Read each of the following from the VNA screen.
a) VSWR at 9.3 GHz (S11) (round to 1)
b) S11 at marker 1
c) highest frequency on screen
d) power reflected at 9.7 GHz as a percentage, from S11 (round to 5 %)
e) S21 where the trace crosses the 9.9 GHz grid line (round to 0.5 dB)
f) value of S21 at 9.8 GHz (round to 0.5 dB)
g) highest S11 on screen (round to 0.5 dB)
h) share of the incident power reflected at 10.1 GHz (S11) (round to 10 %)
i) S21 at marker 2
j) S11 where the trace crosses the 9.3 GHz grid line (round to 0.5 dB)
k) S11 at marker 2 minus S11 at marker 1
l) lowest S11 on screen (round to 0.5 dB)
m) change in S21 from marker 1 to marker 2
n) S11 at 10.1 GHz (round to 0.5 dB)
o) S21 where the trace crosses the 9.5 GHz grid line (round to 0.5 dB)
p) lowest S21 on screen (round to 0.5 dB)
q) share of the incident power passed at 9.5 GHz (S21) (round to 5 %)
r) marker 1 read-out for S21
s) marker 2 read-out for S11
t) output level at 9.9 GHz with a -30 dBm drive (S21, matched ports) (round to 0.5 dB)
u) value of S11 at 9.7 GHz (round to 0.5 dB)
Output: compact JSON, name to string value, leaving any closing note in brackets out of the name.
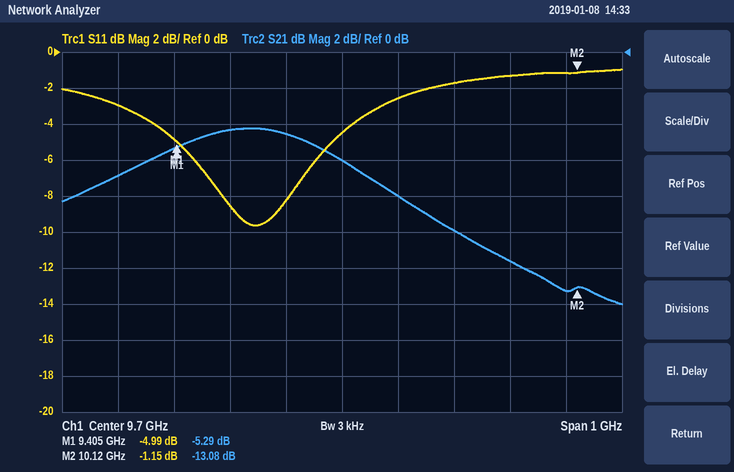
{"VSWR at 9.3 GHz (S11)": "6", "S11 at marker 1": "-4.99 dB", "highest frequency on screen": "10.2 GHz", "power reflected at 9.7 GHz as a percentage, from S11": "35 %", "S21 where the trace crosses the 9.9 GHz grid line": "-10.0 dB", "value of S21 at 9.8 GHz": "-8.0 dB", "highest S11 on screen": "-1.0 dB", "share of the incident power reflected at 10.1 GHz (S11)": "80 %", "S21 at marker 2": "-13.08 dB", "S11 where the trace crosses the 9.3 GHz grid line": "-3.0 dB", "S11 at marker 2 minus S11 at marker 1": "3.84 dB", "lowest S11 on screen": "-9.5 dB", "change in S21 from marker 1 to marker 2": "-7.79 dB", "S11 at 10.1 GHz": "-1.0 dB", "S21 where the trace crosses the 9.5 GHz grid line": "-4.5 dB", "lowest S21 on screen": "-14.0 dB", "share of the incident power passed at 9.5 GHz (S21)": "35 %", "marker 1 read-out for S21": "-5.29 dB", "marker 2 read-out for S11": "-1.15 dB", "output level at 9.9 GHz with a -30 dBm drive (S21, matched ports)": "-40.0 dBm", "value of S11 at 9.7 GHz": "-4.5 dB"}
